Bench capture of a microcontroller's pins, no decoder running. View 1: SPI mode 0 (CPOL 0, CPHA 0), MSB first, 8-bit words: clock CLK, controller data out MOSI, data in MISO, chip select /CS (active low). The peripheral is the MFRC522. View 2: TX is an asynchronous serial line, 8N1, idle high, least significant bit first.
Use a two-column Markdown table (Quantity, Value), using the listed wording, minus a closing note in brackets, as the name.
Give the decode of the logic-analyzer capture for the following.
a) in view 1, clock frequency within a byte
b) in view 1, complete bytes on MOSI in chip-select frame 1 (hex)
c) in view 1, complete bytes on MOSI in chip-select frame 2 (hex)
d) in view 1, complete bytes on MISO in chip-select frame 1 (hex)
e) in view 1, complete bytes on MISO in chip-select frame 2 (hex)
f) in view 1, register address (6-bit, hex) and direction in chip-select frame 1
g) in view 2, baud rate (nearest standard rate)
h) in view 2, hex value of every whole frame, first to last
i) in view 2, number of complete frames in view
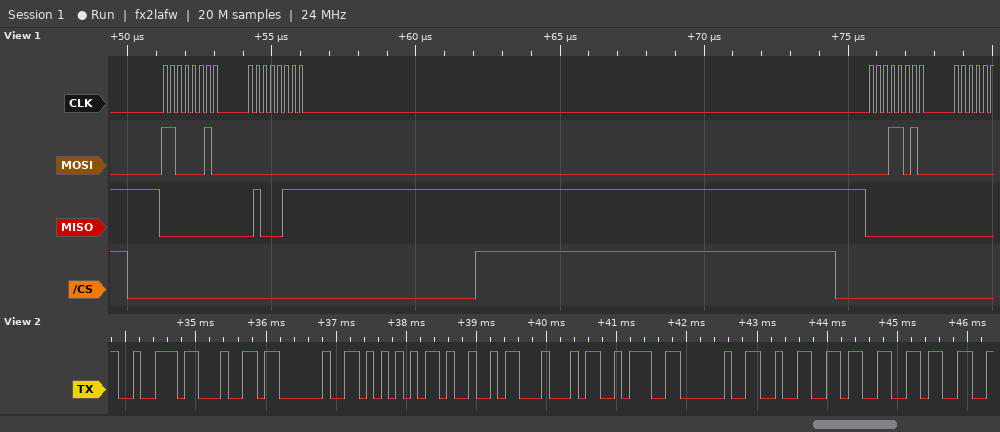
| Quantity | Value |
|---|---|
| in view 1, clock frequency within a byte | 4 MHz |
| in view 1, complete bytes on MOSI in chip-select frame 1 | C2 00 |
| in view 1, complete bytes on MOSI in chip-select frame 2 | 1A |
| in view 1, complete bytes on MISO in chip-select frame 1 | 00 47 |
| in view 1, complete bytes on MISO in chip-select frame 2 | 00 |
| in view 1, register address (6-bit, hex) and direction in chip-select frame 1 | 0x21 read |
| in view 2, baud rate | 9600 baud |
| in view 2, hex value of every whole frame, first to last | 0x72 0x64 0x20 0x55 0x49 0x44 0x3A 0x20 0x32 0x33 0x33 |
| in view 2, number of complete frames in view | 11 |
